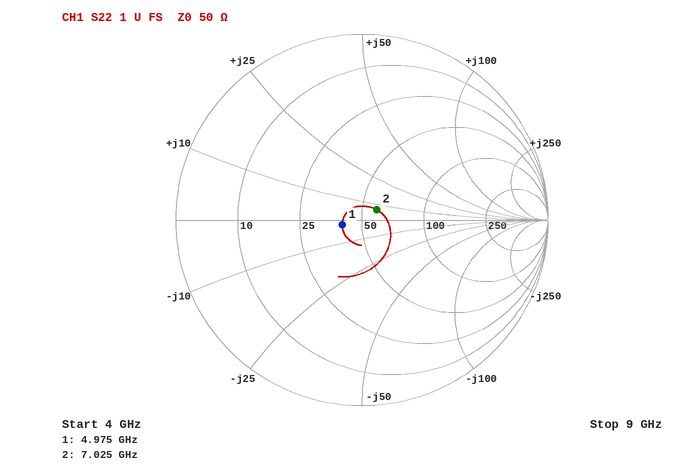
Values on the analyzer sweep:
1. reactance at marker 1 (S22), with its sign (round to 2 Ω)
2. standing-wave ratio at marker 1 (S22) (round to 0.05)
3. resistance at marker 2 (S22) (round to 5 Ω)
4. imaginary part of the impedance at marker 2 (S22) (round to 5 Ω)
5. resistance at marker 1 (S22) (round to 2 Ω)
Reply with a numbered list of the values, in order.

1. -2 Ω
2. 1.25
3. 60 Ω
4. +5 Ω
5. 40 Ω
